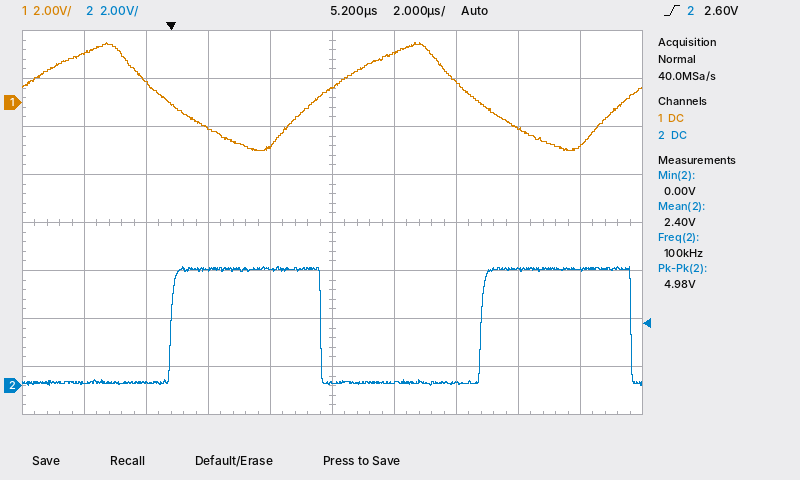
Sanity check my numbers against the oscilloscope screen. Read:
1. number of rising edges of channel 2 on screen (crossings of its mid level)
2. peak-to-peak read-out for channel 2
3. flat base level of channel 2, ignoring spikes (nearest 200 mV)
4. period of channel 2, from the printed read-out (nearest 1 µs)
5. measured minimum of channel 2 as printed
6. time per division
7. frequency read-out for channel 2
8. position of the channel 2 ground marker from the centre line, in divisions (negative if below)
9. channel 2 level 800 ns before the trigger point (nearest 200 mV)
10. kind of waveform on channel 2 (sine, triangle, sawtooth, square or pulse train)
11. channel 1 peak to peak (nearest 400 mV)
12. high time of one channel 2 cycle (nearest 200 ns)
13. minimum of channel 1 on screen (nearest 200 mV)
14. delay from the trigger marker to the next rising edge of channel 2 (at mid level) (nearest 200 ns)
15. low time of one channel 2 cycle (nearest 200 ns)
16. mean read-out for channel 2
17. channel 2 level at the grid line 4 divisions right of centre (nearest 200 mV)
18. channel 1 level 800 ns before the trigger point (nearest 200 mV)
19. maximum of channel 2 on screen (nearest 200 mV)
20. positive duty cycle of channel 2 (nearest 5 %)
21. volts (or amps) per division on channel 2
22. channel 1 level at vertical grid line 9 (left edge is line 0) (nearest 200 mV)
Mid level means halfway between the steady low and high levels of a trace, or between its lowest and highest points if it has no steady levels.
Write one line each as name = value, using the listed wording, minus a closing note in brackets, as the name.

number of rising edges of channel 2 on screen = 2
peak-to-peak read-out for channel 2 = 4.98 V
flat base level of channel 2, ignoring spikes = 200 mV
period of channel 2, from the printed read-out = 10 µs
measured minimum of channel 2 as printed = 0.00 V
time per division = 2 µs
frequency read-out for channel 2 = 100 kHz
position of the channel 2 ground marker from the centre line, in divisions = -3.4 div
channel 2 level 800 ns before the trigger point = 200 mV
kind of waveform on channel 2 = square
channel 1 peak to peak = 4.4 V
high time of one channel 2 cycle = 4.8 µs
minimum of channel 1 on screen = -2.0 V
delay from the trigger marker to the next rising edge of channel 2 (at mid level) = 10.0 µs
low time of one channel 2 cycle = 5.2 µs
mean read-out for channel 2 = 2.40 V
channel 2 level at the grid line 4 divisions right of centre = 4.8 V
channel 1 level 800 ns before the trigger point = 800 mV
maximum of channel 2 on screen = 5.0 V
positive duty cycle of channel 2 = 50 %
volts (or amps) per division on channel 2 = 2 V
channel 1 level at vertical grid line 9 (left edge is line 0) = -1.8 V
